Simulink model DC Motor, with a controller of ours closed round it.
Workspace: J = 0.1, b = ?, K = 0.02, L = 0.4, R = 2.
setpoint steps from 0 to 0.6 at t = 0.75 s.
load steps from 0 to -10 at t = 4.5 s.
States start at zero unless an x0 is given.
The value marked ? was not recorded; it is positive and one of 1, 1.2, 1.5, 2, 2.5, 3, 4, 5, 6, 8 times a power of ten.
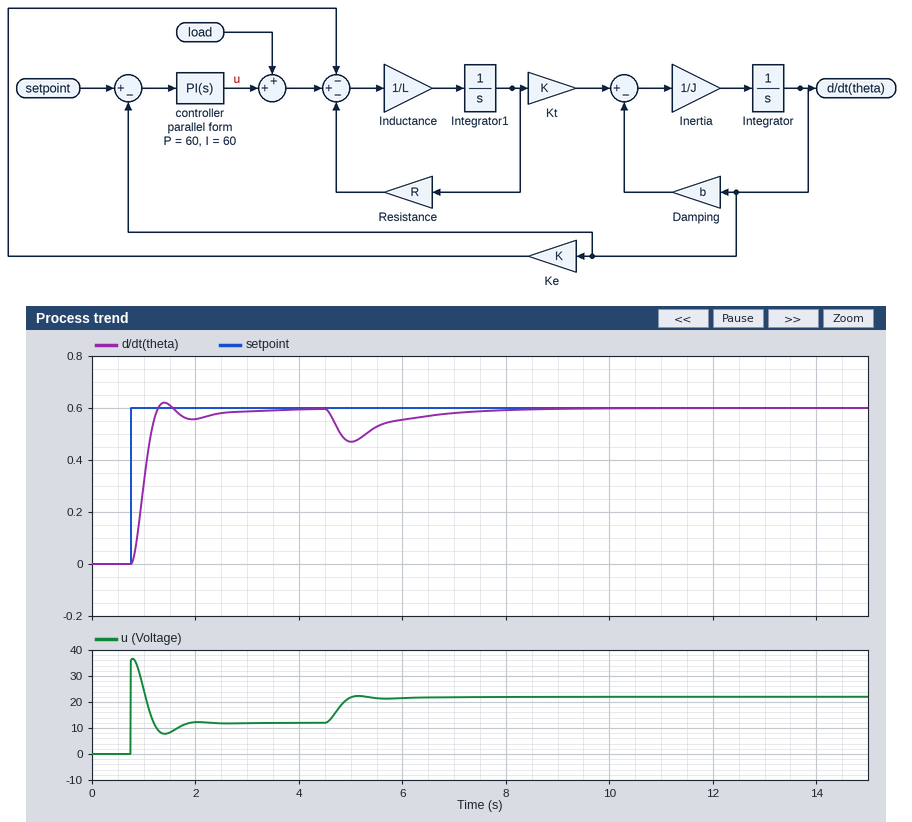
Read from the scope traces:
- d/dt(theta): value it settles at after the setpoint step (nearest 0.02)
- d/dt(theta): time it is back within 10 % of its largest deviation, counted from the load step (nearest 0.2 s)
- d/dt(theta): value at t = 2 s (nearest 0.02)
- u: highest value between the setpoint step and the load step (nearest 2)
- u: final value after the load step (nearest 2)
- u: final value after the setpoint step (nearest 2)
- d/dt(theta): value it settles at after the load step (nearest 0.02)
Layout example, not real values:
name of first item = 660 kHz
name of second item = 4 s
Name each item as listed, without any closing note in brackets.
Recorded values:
d/dt(theta): value it settles at after the setpoint step = 0.60
d/dt(theta): time it is back within 10 % of its largest deviation, counted from the load step = 3.0 s
d/dt(theta): value at t = 2 s = 0.56
u: highest value between the setpoint step and the load step = 36
u: final value after the load step = 22
u: final value after the setpoint step = 12
d/dt(theta): value it settles at after the load step = 0.60
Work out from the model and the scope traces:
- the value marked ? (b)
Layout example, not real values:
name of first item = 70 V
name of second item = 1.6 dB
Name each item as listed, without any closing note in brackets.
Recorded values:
the value marked ? = 0.2
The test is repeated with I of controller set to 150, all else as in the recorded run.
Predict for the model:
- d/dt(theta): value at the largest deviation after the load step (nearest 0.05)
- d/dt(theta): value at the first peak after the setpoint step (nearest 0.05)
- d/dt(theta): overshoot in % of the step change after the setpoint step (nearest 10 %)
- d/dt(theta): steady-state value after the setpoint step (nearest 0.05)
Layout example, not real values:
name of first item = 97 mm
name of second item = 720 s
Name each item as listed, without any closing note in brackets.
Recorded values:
d/dt(theta): value at the largest deviation after the load step = 0.50
d/dt(theta): value at the first peak after the setpoint step = 0.75
d/dt(theta): overshoot in % of the step change after the setpoint step = 30 %
d/dt(theta): steady-state value after the setpoint step = 0.60
